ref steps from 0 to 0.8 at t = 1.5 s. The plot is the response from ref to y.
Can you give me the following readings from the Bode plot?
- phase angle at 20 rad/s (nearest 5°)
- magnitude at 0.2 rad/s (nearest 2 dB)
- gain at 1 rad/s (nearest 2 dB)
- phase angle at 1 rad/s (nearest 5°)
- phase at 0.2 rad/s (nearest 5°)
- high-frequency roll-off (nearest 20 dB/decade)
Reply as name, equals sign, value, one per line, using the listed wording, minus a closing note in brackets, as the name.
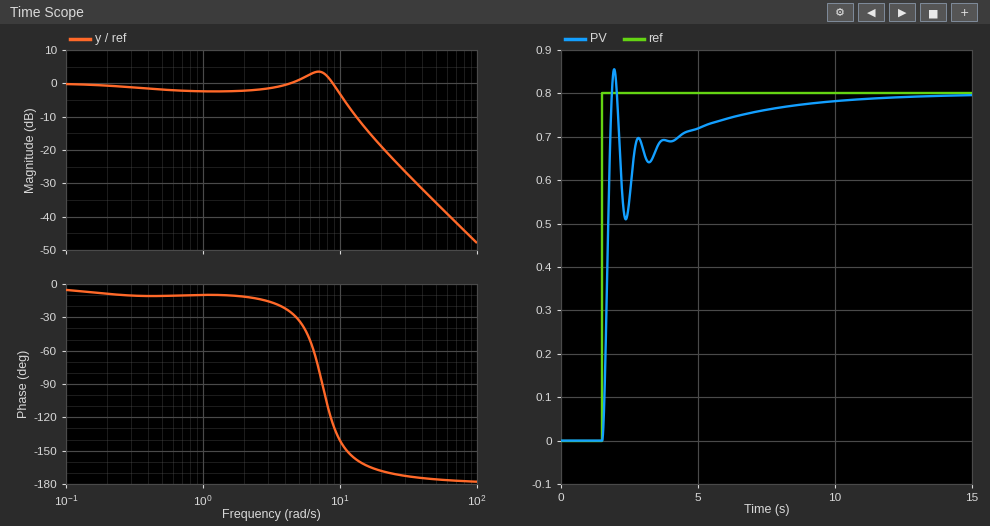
phase angle at 20 rad/s = -170°
magnitude at 0.2 rad/s = 0 dB
gain at 1 rad/s = -2 dB
phase angle at 1 rad/s = -10°
phase at 0.2 rad/s = -10°
high-frequency roll-off = -40 dB/decade
